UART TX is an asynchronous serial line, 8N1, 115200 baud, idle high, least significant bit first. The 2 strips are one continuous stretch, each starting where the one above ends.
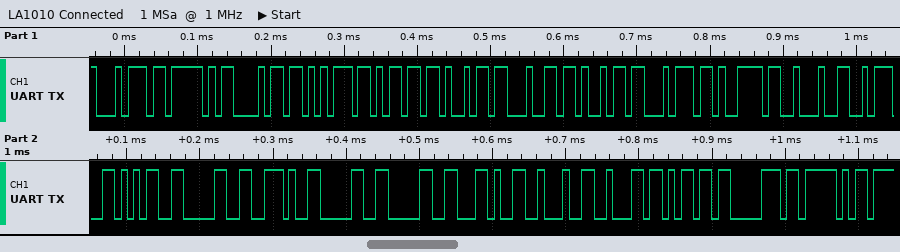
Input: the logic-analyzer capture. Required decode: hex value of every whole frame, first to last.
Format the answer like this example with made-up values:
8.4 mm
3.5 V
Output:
0x74 0x5F 0x68 0x75 0x6D 0x69 0x64 0x69 0x74 0x79 0x22 0x3A 0x35 0x30 0x2E 0x30 0x30 0x2C 0x22 0x62 0x6D 0x70 0x5F
